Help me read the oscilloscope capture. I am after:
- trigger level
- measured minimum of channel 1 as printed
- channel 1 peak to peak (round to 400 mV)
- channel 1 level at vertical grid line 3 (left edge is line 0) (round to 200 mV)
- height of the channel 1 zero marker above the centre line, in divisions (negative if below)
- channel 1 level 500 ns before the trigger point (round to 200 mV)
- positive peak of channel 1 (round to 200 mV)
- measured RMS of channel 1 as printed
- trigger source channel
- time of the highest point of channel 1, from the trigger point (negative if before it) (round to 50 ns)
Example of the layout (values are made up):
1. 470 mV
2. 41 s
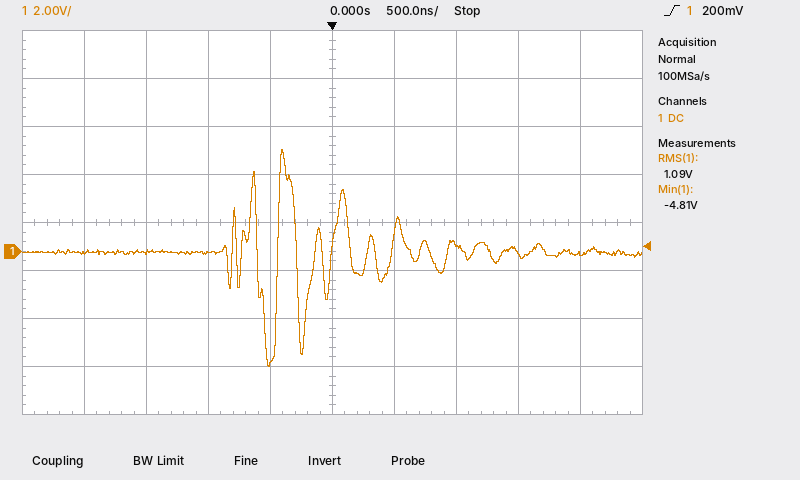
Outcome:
1. 200 mV
2. -4.81 V
3. 9.2 V
4. 0.0 V
5. -0.6 div
6. -4.6 V
7. 4.2 V
8. 1.09 V
9. channel 1
10. -400 ns
